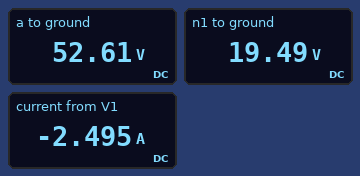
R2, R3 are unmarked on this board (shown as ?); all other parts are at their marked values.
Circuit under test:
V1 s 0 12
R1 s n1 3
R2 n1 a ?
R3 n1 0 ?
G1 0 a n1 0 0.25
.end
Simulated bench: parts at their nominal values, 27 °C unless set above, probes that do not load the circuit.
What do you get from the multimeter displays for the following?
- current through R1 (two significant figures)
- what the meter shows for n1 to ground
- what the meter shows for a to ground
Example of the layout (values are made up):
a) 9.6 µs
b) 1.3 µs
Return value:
a) 2.5 A
b) 19.49 V
c) 52.61 V
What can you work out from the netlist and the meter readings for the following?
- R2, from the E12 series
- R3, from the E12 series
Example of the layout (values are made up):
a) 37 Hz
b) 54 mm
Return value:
a) 6.8 Ω
b) 8.2 Ω
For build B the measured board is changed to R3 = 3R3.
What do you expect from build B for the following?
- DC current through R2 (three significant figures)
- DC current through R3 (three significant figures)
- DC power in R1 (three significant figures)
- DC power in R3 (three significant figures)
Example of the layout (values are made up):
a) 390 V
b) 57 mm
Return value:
a) 2.59 A
b) 3.14 A
c) 904 mW
d) 32.5 W
